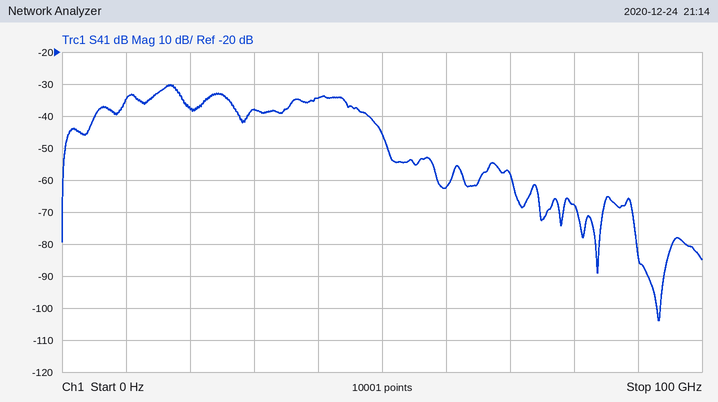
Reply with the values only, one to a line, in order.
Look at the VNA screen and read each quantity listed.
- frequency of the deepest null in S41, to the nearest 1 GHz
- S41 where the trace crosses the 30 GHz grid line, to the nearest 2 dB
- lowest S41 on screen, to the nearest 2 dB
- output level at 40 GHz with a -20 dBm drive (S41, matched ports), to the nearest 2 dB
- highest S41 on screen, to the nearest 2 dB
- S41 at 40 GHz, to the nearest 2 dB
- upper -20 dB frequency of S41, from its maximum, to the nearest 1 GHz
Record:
93 GHz
-38 dB
-104 dB
-54 dBm
-30 dB
-34 dB
51 GHz
